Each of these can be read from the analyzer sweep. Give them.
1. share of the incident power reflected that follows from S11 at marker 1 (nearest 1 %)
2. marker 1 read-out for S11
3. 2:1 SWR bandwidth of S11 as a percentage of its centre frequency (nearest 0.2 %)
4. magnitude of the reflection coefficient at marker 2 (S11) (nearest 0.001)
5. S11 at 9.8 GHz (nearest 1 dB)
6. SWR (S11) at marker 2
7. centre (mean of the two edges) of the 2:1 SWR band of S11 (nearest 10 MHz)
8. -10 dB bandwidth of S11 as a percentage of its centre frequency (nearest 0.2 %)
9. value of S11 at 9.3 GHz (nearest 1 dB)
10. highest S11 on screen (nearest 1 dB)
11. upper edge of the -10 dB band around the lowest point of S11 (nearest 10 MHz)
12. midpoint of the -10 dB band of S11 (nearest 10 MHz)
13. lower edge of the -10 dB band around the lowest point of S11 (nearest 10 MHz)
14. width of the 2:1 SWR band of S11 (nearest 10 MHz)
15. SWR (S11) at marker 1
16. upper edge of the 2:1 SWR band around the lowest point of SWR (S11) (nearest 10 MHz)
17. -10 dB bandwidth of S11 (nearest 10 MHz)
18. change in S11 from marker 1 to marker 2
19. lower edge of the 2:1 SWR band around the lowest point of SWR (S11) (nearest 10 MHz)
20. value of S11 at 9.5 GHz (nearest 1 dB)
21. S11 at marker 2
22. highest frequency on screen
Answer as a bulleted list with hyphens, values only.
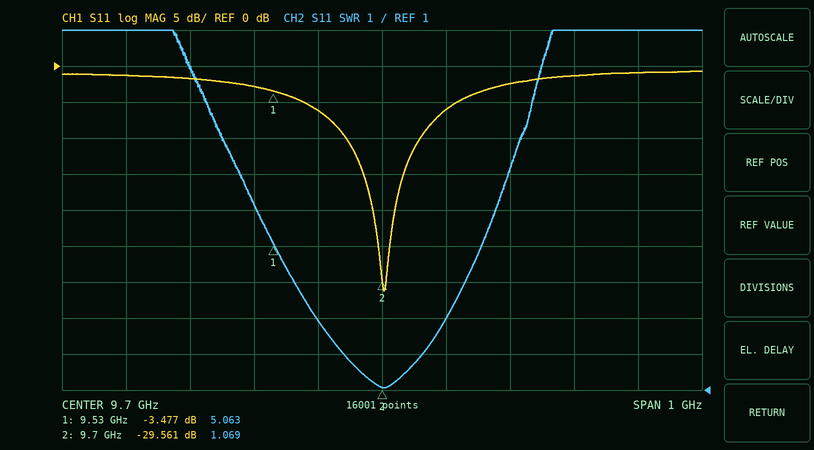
- 45 %
- -3.477 dB
- 1.2 %
- 0.033
- -6 dB
- 1.069
- 9.70 GHz
- 1.2 %
- -1 dB
- -1 dB
- 9.76 GHz
- 9.70 GHz
- 9.64 GHz
- 120 MHz
- 5.063
- 9.76 GHz
- 120 MHz
- -26.084 dB
- 9.64 GHz
- -3 dB
- -29.561 dB
- 10.2 GHz
